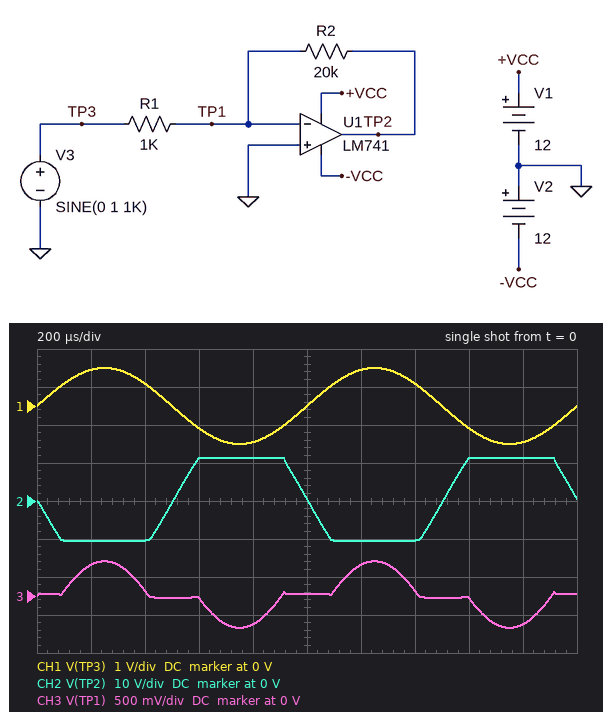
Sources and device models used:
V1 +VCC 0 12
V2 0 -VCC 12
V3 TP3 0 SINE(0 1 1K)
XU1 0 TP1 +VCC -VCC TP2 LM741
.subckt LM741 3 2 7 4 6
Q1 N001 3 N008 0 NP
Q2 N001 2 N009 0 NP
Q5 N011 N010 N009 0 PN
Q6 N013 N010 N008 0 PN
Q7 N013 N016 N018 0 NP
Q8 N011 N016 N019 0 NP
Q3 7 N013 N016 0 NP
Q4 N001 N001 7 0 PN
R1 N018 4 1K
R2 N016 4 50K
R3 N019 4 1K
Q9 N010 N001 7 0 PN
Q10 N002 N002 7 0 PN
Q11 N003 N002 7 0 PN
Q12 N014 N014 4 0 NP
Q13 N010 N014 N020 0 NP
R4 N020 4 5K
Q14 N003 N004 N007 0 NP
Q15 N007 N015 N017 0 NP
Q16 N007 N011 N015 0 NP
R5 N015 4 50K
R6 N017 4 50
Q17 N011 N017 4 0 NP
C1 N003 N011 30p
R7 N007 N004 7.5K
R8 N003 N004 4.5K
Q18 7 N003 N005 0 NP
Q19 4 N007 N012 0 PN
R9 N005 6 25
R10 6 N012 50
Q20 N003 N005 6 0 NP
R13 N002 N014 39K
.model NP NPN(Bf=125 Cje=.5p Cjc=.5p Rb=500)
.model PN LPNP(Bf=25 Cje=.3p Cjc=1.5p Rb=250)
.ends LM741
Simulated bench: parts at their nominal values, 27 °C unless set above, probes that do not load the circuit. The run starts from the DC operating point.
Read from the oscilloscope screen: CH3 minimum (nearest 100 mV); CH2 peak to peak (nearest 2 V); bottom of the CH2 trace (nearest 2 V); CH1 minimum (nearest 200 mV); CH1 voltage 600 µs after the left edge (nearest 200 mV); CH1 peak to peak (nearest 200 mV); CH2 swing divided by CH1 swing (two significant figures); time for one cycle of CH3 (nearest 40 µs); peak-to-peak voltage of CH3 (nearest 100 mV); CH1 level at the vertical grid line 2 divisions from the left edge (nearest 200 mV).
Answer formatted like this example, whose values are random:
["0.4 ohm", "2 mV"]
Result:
["-400 mV", "22 V", "-10 V", "-1.0 V", "-600 mV", "2.0 V", "11", "1.00 ms", "900 mV", "600 mV"]
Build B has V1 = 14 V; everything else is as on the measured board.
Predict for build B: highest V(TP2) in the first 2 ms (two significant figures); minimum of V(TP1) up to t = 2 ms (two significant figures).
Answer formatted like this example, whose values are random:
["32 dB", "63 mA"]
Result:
["13 V", "-320 mV"]
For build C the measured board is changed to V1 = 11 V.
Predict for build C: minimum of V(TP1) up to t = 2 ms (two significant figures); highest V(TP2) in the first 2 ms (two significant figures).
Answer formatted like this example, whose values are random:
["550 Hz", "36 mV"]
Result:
["-470 mV", "10 V"]
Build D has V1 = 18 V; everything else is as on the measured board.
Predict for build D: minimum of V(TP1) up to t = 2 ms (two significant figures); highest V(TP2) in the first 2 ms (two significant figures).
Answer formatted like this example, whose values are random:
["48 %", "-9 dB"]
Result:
["-130 mV", "17 V"]
